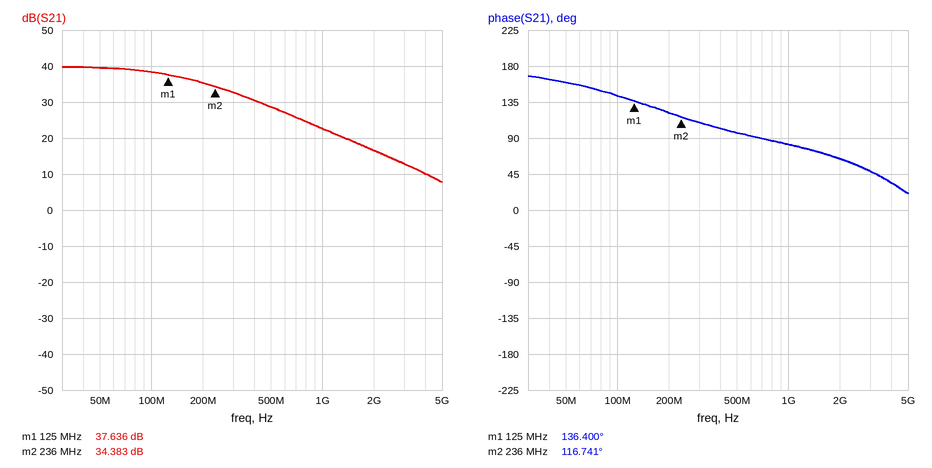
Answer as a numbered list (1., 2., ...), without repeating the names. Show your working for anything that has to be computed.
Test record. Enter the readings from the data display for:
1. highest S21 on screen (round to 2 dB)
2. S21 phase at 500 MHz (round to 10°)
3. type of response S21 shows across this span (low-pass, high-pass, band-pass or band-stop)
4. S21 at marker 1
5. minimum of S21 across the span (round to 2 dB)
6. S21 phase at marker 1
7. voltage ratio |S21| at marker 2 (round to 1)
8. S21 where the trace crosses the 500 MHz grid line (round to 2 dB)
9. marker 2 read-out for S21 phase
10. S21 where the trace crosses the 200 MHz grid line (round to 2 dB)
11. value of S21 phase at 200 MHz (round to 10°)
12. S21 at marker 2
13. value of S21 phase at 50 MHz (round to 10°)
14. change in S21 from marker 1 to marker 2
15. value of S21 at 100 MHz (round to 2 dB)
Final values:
1. 40 dB
2. 100°
3. low-pass
4. 37.636 dB
5. 8 dB
6. 136.400°
7. 10^(34.383/20) ≈ 52
8. 28 dB
9. 116.741°
10. 36 dB
11. 120°
12. 34.383 dB
13. 160°
14. 34.383 − (37.636) = -3.253 dB
15. 38 dB
